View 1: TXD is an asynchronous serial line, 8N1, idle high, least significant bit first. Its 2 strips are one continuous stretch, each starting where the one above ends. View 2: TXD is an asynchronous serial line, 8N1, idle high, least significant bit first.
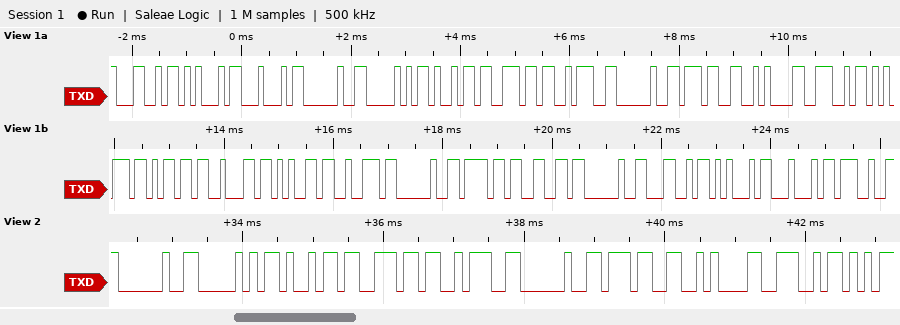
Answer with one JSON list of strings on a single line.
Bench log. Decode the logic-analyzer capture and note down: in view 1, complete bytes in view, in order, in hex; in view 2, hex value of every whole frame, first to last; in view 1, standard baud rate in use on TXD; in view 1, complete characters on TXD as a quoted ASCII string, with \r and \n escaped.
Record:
["4C 45 44 20 50 69 6E 3A 20 37 0A 4E 75 6D 62 65 72 20 6F 66 20 4C 45 44 27", "20 50 69 6E 3A 20 37 0A 4E", "9600 baud", "\"LED Pin: 7\\nNumber of LED'\""]
